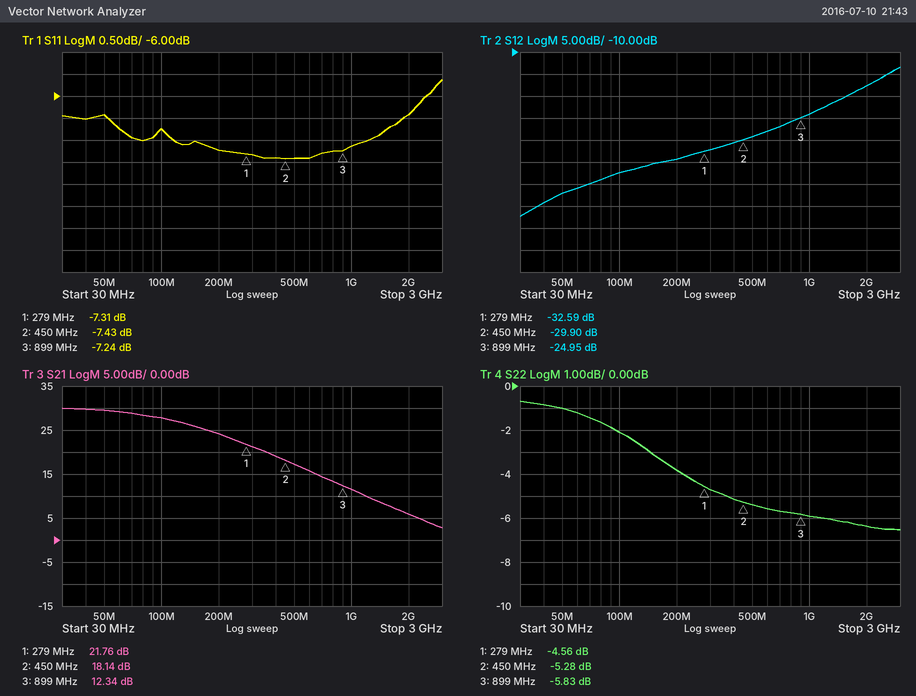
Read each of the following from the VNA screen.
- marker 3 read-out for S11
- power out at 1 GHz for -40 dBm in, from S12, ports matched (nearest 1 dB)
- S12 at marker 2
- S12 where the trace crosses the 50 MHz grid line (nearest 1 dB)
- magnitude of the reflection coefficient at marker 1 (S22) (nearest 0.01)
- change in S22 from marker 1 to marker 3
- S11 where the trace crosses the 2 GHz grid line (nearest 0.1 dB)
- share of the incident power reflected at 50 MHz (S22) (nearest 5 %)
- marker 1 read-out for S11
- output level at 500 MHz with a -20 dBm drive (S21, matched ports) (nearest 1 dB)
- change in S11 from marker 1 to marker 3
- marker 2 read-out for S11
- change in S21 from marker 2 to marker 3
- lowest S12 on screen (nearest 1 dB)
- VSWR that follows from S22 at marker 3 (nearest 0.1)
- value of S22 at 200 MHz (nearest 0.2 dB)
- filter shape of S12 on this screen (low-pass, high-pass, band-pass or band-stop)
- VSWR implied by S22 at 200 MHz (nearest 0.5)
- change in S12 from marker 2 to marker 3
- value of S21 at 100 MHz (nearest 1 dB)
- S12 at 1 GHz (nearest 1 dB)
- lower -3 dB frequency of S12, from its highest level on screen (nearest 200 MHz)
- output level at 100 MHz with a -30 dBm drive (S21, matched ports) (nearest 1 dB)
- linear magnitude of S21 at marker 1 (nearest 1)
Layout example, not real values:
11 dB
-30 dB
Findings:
-7.24 dB
-64 dBm
-29.90 dB
-42 dB
0.59
-1.27 dB
-6.4 dB
80 %
-7.31 dB
-3 dBm
0.07 dB
-7.43 dB
-5.80 dB
-47 dB
3.1
-3.8 dB
high-pass
4.5
4.95 dB
28 dB
-24 dB
2.2 GHz
-2 dBm
12
